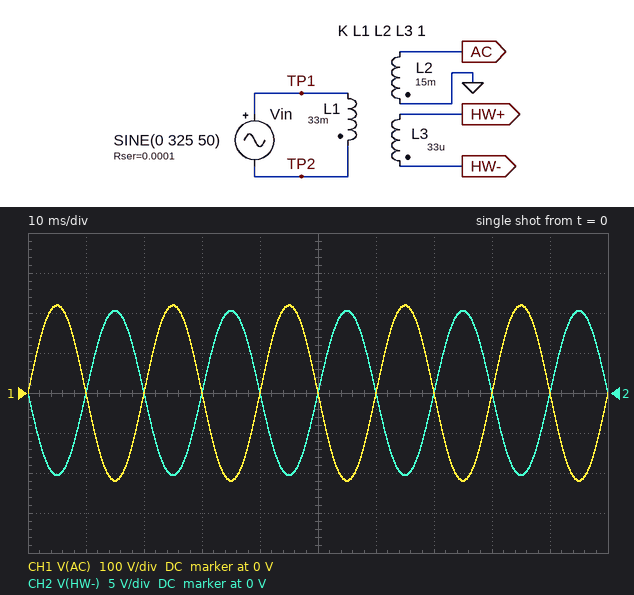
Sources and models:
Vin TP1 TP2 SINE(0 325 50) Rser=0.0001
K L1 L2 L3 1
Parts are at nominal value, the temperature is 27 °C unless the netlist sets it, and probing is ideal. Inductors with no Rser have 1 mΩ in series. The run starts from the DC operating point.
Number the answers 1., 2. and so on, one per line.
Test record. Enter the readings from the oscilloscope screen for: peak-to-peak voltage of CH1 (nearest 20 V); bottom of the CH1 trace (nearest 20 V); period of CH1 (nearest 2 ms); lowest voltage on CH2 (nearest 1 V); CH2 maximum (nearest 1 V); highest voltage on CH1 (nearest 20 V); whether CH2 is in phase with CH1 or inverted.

1. 440 V
2. -220 V
3. 20 ms
4. -10 V
5. 10 V
6. 220 V
7. inverted
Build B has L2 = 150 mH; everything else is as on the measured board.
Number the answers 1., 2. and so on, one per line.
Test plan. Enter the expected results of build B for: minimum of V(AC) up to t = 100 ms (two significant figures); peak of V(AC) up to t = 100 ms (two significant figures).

1. -690 V
2. 690 V
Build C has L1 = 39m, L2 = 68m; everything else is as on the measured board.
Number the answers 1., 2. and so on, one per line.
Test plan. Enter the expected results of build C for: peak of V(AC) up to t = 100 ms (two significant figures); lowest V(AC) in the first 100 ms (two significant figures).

1. 430 V
2. -430 V
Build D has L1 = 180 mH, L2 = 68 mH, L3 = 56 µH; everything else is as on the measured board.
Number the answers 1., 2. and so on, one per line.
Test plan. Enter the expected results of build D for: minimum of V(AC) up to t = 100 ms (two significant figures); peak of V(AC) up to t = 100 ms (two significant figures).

1. -200 V
2. 200 V
